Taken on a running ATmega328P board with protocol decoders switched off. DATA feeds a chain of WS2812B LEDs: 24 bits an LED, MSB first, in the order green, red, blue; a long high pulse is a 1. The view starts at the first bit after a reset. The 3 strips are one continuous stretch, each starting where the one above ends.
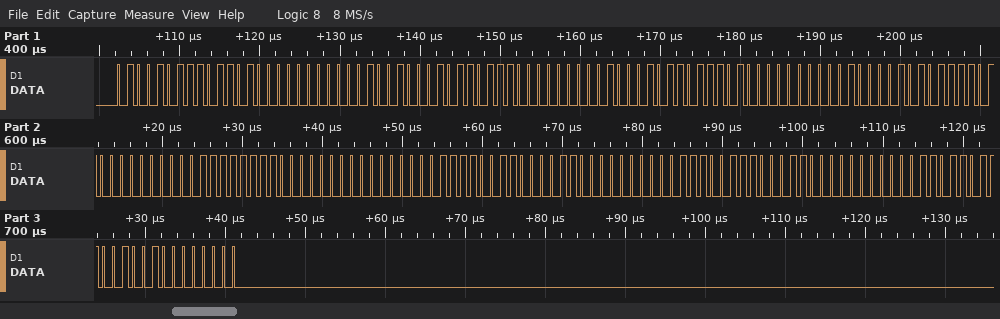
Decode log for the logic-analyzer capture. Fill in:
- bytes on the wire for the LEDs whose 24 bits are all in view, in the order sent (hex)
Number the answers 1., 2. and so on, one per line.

1. 4B B4 00 48 B7 00 45 BA 00 42 BD 00 3F C0 00 3C C3 00 39 C6 00 36 C9 00
